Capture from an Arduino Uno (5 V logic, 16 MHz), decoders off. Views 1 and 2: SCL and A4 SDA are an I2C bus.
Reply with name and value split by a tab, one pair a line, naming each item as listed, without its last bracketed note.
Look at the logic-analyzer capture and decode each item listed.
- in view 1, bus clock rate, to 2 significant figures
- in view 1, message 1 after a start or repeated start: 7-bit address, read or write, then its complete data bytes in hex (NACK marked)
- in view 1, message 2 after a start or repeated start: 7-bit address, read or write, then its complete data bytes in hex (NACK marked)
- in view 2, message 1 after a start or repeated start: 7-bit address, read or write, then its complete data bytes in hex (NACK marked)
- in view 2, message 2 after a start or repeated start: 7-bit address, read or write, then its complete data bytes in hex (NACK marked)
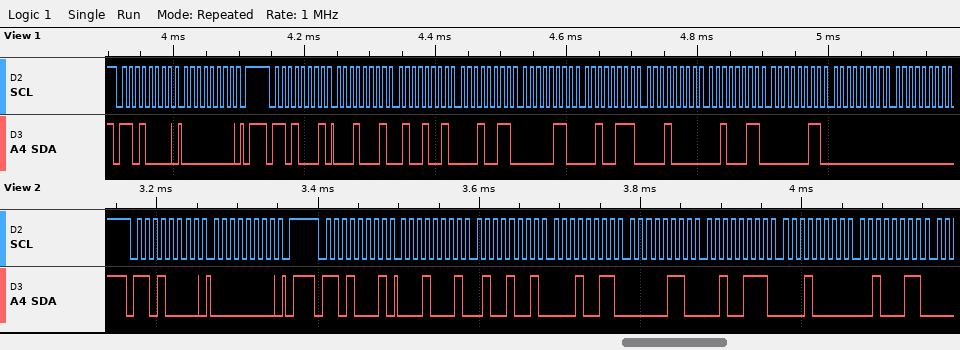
in view 1, bus clock rate, to 2 significant figures	100 kHz
in view 1, message 1 after a start or repeated start: 7-bit address, read or write, then its complete data bytes in hex	0x68 write: 00
in view 1, message 2 after a start or repeated start: 7-bit address, read or write, then its complete data bytes in hex	0x68 read: 11 49 13 06 27 10 23 03 00 00
in view 2, message 1 after a start or repeated start: 7-bit address, read or write, then its complete data bytes in hex	0x68 write: 00
in view 2, message 2 after a start or repeated start: 7-bit address, read or write, then its complete data bytes in hex	0x68 read: 11 49 13 06 27 10 23
